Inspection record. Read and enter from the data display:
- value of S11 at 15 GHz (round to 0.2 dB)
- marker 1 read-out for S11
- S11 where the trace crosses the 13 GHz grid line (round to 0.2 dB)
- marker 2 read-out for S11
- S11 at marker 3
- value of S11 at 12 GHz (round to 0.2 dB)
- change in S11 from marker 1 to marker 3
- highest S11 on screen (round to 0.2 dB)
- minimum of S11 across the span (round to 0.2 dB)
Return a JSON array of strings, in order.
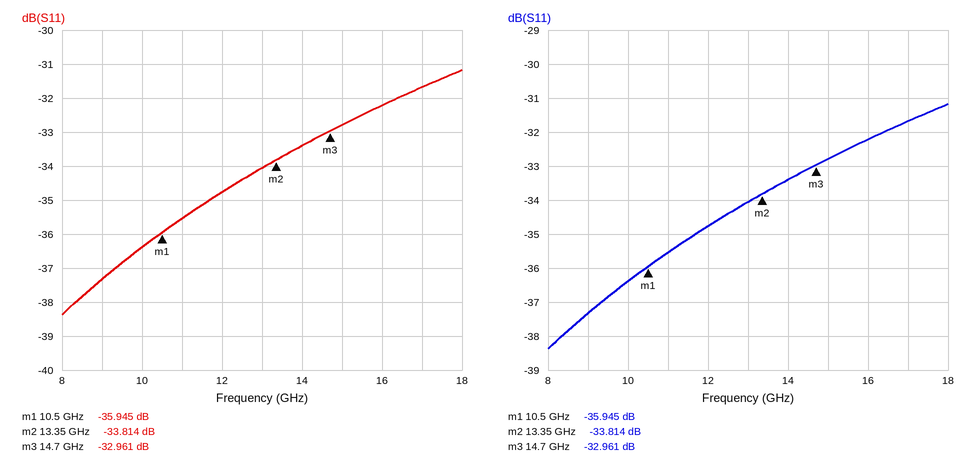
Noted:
["-32.8 dB", "-35.945 dB", "-34.0 dB", "-33.814 dB", "-32.961 dB", "-34.8 dB", "2.984 dB", "-31.2 dB", "-38.4 dB"]
